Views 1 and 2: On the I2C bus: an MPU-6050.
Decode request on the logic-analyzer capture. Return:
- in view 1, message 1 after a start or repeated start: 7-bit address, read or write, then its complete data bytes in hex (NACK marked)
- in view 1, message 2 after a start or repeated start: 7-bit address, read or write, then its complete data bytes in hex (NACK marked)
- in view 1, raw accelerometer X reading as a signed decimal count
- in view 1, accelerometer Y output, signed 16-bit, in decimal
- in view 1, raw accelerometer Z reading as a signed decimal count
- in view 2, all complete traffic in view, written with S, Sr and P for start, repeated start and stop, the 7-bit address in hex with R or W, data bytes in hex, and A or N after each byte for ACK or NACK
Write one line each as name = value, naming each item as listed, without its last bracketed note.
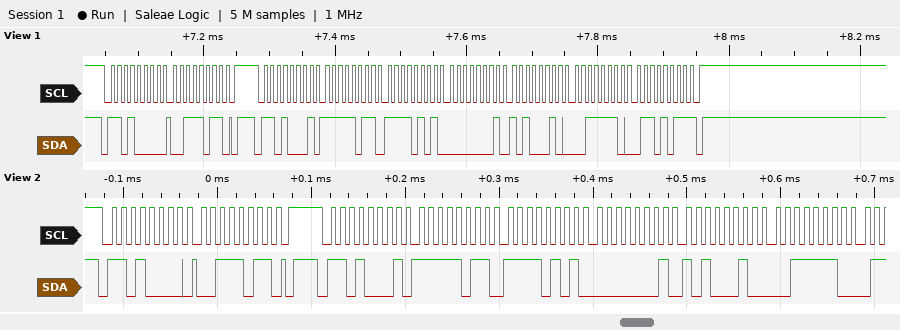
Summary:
in view 1, message 1 after a start or repeated start: 7-bit address, read or write, then its complete data bytes in hex = 0x68 write: 3B
in view 1, message 2 after a start or repeated start: 7-bit address, read or write, then its complete data bytes in hex = 0x68 read: FB F5 01 A2 3E 6B NACK
in view 1, raw accelerometer X reading as a signed decimal count = -1035
in view 1, accelerometer Y output, signed 16-bit, in decimal = 418
in view 1, raw accelerometer Z reading as a signed decimal count = 15979
in view 2, all complete traffic in view, written with S, Sr and P for start, repeated start and stop, the 7-bit address in hex with R or W, data bytes in hex, and A or N after each byte for ACK or NACK = S 68W A 3B A P S 68R A FB A F5 A 01 A A2 A 3E A
